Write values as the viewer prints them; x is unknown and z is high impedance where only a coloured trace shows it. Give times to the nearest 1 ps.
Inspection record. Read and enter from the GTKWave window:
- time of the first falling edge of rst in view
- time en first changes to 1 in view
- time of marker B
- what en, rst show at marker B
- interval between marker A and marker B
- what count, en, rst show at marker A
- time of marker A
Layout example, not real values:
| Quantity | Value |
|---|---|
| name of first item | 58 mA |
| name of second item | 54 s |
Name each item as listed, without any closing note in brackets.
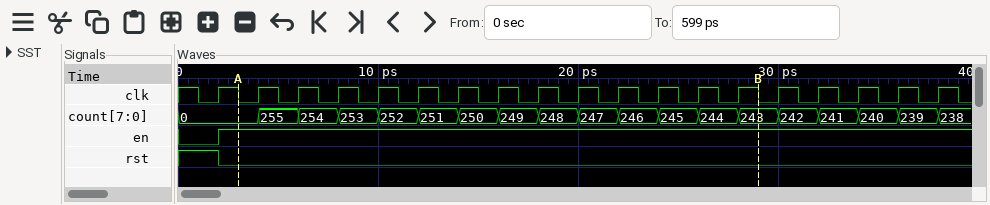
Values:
| Quantity | Value |
|---|---|
| time of the first falling edge of rst in view | 2 ps |
| time en first changes to 1 in view | 2 ps |
| time of marker B | 29 ps |
| what en, rst show at marker B | en=1, rst=0 |
| interval between marker A and marker B | 26 ps |
| what count, en, rst show at marker A | count=0, en=1, rst=0 |
| time of marker A | 3 ps |
